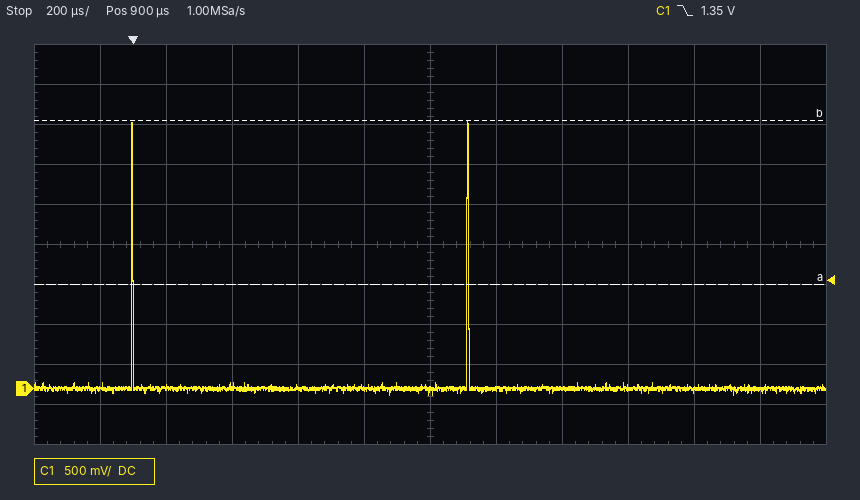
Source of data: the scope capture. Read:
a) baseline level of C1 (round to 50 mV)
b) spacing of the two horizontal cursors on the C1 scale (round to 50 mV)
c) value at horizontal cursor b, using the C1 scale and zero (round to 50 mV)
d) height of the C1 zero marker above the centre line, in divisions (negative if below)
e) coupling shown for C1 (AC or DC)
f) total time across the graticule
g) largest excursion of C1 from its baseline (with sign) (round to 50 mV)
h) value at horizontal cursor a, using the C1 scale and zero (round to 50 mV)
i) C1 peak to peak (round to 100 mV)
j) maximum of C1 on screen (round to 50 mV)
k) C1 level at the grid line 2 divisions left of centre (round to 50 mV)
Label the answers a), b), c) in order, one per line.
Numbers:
a) 0 mV
b) 2.05 V
c) 3.35 V
d) -3.6 div
e) DC
f) 2.4 ms
g) +3.35 V
h) 1.30 V
i) 3.40 V
j) 3.35 V
k) 0 mV
